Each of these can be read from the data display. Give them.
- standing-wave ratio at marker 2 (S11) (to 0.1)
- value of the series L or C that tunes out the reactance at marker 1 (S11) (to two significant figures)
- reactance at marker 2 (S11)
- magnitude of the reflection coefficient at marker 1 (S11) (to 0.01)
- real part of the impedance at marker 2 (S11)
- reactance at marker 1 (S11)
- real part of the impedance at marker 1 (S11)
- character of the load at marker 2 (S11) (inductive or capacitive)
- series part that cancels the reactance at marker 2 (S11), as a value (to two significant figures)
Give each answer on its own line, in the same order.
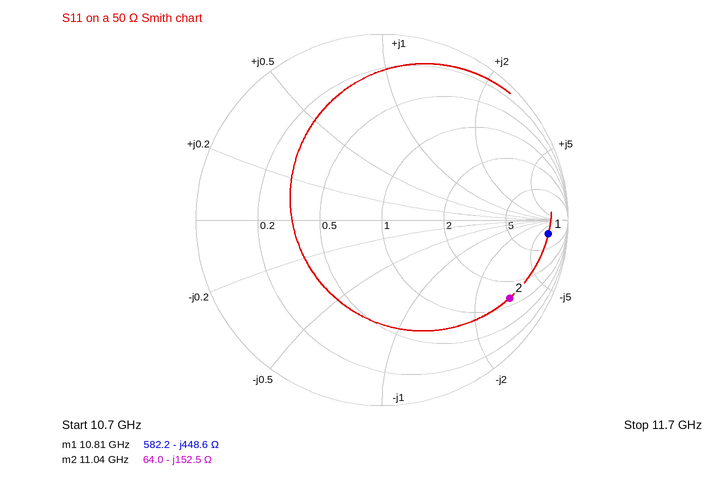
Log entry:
9.2
6.6 nH
-152.5 Ω
0.90
64.0 Ω
-448.6 Ω
582.2 Ω
capacitive
2.2 nH
